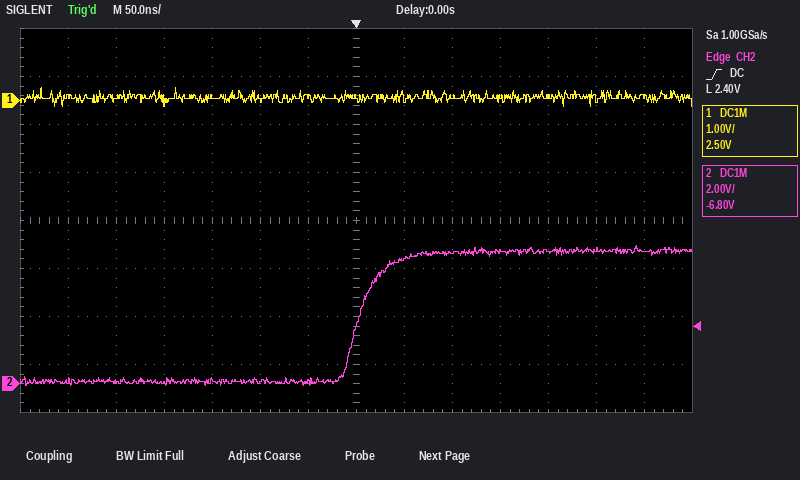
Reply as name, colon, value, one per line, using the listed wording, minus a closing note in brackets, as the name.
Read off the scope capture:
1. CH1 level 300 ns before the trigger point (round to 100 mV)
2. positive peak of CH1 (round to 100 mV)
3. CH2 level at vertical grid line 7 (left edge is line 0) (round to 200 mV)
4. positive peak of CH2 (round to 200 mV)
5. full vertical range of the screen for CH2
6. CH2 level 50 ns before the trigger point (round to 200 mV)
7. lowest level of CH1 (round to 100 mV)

CH1 level 300 ns before the trigger point: 100 mV
positive peak of CH1: 300 mV
CH2 level at vertical grid line 7 (left edge is line 0): 2.4 V
positive peak of CH2: 5.8 V
full vertical range of the screen for CH2: 16 V
CH2 level 50 ns before the trigger point: 0.0 V
lowest level of CH1: -100 mV
